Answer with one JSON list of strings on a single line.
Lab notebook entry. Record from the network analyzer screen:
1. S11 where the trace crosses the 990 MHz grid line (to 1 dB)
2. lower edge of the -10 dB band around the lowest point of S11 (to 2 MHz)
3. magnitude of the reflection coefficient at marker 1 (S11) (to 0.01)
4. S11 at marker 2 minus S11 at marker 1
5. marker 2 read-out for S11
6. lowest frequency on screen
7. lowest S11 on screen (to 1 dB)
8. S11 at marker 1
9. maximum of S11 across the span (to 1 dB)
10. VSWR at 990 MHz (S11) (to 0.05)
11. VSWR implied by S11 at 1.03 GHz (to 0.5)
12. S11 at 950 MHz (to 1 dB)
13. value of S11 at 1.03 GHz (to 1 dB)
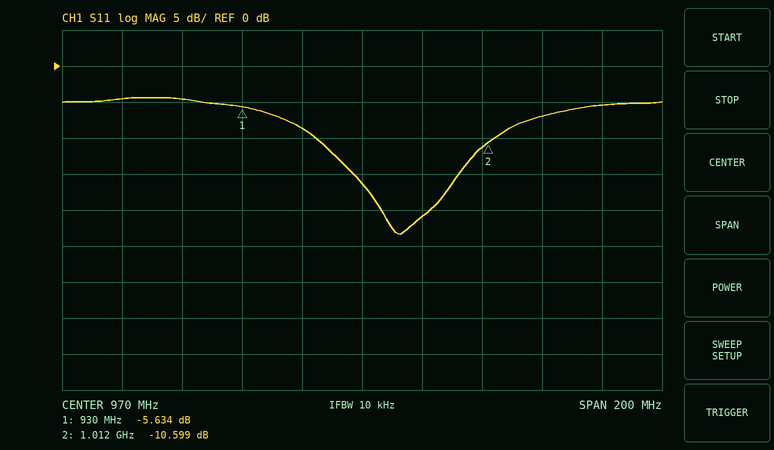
["-21 dB", "954 MHz", "0.52", "-4.965 dB", "-10.599 dB", "870 MHz", "-23 dB", "-5.634 dB", "-4 dB", "1.20", "2.5", "-9 dB", "-7 dB"]
